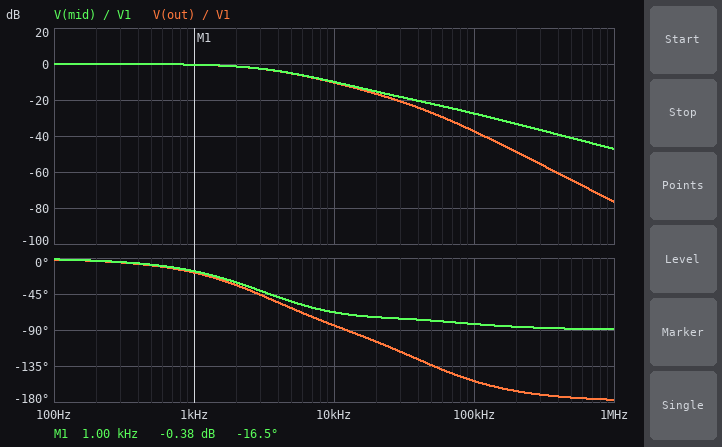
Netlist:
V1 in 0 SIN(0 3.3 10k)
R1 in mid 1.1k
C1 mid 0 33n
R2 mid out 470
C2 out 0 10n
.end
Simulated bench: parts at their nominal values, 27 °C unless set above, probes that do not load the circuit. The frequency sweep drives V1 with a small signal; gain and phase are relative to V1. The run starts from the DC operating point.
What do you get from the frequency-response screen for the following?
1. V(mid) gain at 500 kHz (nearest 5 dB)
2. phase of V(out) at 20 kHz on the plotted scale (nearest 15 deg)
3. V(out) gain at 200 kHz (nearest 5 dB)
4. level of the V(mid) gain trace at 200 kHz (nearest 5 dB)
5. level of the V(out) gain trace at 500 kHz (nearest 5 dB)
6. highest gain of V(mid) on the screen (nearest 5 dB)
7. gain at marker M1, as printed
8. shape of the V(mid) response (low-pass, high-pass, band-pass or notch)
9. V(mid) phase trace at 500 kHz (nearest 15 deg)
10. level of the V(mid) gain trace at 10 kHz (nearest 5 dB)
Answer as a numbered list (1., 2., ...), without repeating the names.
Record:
1. -40 dB
2. -105 deg
3. -50 dB
4. -35 dB
5. -65 dB
6. 0 dB
7. -0.38 dB
8. low-pass
9. -90 deg
10. -10 dB
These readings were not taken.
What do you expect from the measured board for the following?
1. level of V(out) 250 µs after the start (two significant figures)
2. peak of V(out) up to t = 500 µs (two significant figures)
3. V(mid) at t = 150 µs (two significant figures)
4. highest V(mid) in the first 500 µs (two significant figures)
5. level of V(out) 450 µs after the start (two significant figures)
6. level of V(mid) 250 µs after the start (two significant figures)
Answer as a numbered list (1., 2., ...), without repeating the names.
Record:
1. 1.0 V
2. 1.4 V
3. 1.0 V
4. 1.4 V
5. 1.0 V
6. 980 mV
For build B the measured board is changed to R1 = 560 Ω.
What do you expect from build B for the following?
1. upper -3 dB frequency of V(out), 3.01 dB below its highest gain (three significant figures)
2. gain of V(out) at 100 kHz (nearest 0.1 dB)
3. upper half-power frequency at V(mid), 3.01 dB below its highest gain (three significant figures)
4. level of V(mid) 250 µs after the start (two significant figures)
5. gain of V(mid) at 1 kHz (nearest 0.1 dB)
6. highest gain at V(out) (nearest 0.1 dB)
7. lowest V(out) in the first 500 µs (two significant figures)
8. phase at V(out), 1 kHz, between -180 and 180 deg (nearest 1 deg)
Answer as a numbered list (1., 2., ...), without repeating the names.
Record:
1. 6.17 kHz
2. -31.6 dB
3. 6.38 kHz
4. 1.4 V
5. -0.1 dB
6. 0 dB
7. -1.7 V
8. -10 deg
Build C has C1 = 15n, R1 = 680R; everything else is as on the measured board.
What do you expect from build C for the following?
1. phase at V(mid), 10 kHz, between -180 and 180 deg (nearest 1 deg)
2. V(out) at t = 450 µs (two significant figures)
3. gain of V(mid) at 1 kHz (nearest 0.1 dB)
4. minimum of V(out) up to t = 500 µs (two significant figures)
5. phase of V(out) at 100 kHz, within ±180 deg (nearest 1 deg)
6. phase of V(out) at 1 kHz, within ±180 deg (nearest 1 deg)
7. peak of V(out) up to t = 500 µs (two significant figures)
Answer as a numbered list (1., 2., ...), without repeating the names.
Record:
1. -43 deg
2. 1.8 V
3. -0.1 dB
4. -2.1 V
5. -143 deg
6. -8 deg
7. 2.3 V
